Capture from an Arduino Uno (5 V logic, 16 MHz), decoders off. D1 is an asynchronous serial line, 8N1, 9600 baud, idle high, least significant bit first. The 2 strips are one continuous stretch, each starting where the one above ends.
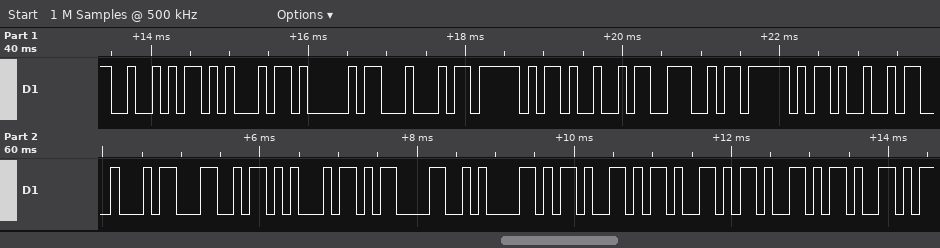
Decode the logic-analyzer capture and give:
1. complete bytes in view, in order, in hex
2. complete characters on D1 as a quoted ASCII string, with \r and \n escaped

0x52 0x45 0x41 0x44 0x5F 0x49 0x4E 0x5F 0x49 0x44 0x4C 0x45 0x0D 0x0A 0x2D 0x2D 0x2D 0x2D
"READ_IN_IDLE\r\n----"
